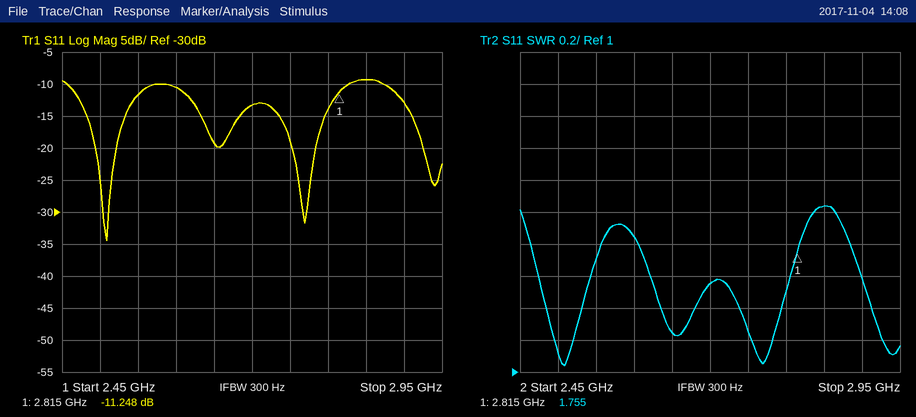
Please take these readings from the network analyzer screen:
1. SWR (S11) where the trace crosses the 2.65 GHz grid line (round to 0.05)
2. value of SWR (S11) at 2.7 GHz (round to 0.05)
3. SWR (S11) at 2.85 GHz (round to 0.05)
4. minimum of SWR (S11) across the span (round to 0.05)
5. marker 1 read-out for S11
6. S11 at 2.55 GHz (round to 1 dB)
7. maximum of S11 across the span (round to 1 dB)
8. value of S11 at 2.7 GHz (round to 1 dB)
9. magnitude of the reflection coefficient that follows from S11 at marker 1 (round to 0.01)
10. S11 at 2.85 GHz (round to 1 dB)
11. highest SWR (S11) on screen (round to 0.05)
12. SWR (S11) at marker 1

1.25
1.55
2.05
1.05
-11.248 dB
-12 dB
-9 dB
-13 dB
0.27
-9 dB
2.05
1.755
